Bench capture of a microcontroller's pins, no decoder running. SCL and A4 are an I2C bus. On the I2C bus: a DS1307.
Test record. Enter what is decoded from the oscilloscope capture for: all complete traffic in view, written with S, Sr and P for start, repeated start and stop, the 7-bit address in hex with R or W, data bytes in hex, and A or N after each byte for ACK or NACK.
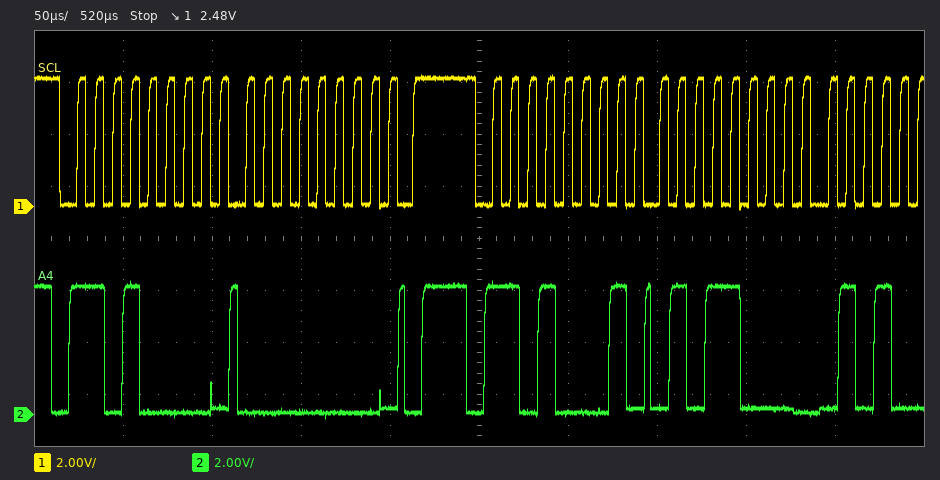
S 68W A 00 A P S 68R A 58 A
